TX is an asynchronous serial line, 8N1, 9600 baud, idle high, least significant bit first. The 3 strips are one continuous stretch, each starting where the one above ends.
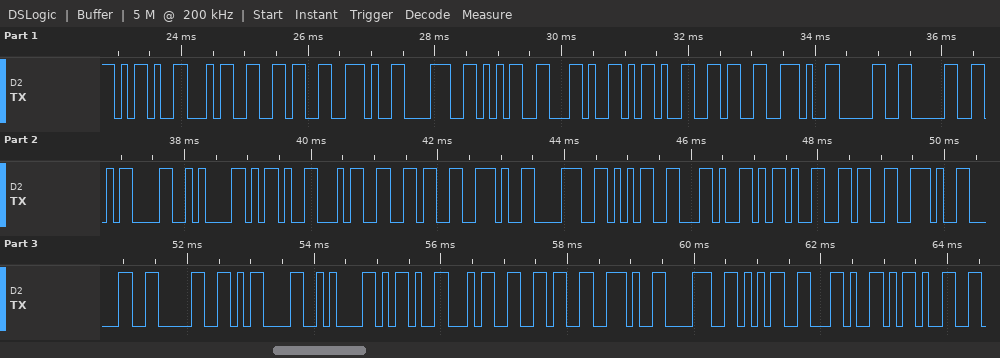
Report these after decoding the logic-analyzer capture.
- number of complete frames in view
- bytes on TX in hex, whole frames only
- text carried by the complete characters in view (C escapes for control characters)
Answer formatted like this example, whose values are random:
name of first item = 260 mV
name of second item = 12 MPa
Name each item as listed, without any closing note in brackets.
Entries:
number of complete frames in view = 36
bytes on TX in hex, whole frames only = 0x2D 0x34 0x36 0x2E 0x38 0x35 0x2C 0x2D 0x36 0x2E 0x30 0x30 0x0D 0x0A 0x2D 0x34 0x36 0x2E 0x38 0x35 0x2C 0x2D 0x36 0x2E 0x30 0x30 0x0D 0x0A 0x2D 0x34 0x36 0x2E 0x38 0x35 0x2C 0x2D
text carried by the complete characters in view = "-46.85,-6.00\r\n-46.85,-6.00\r\n-46.85,-"
